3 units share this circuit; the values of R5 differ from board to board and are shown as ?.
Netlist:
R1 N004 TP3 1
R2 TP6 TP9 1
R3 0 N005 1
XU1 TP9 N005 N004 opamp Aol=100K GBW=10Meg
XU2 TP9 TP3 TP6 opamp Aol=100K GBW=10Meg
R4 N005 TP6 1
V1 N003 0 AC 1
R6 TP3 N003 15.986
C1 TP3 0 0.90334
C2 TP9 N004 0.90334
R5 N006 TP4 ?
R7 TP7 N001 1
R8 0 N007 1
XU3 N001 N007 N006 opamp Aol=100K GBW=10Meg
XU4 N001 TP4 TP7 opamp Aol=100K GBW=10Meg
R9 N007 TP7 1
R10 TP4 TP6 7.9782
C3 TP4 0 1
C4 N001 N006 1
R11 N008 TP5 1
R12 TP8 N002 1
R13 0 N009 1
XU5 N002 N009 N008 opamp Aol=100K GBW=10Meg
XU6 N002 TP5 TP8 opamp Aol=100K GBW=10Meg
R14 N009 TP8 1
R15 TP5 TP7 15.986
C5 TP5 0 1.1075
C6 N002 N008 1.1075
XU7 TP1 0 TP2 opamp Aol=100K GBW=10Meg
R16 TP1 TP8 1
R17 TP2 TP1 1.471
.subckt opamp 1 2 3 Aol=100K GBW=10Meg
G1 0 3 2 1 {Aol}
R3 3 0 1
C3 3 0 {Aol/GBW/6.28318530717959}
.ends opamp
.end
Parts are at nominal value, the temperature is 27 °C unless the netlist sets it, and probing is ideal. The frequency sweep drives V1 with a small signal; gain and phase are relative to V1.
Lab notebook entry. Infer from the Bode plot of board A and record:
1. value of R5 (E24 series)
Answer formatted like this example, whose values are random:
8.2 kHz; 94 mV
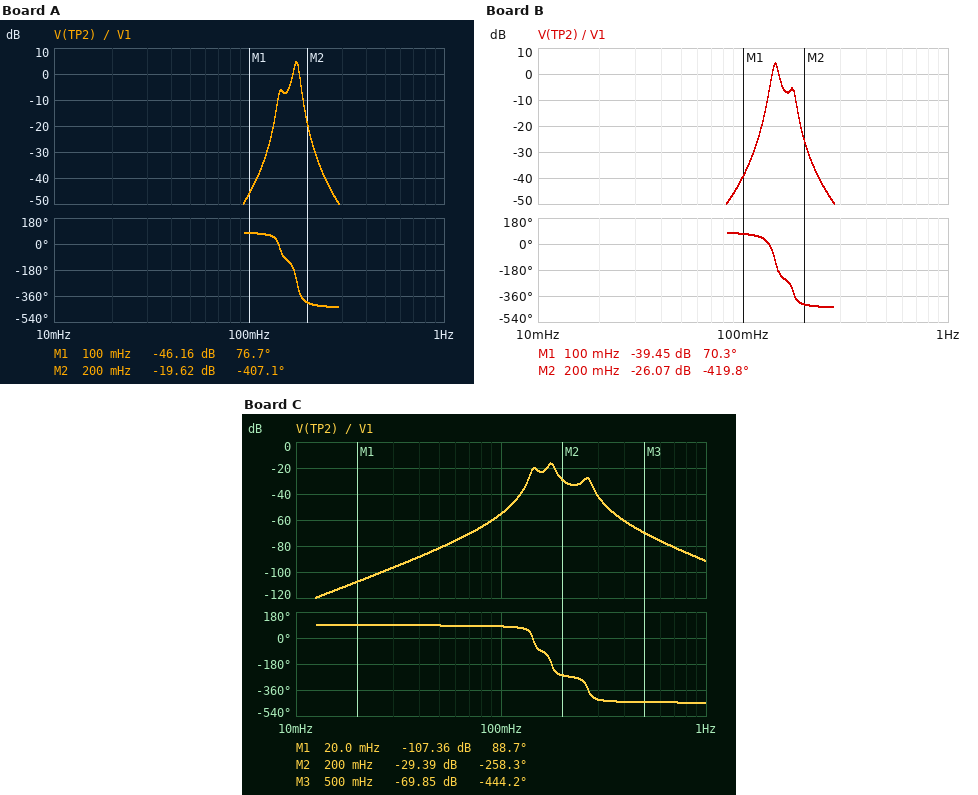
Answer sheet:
0.82 Ω
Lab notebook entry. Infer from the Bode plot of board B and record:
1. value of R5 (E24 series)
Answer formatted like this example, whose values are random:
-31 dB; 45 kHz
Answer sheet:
1.3 Ω
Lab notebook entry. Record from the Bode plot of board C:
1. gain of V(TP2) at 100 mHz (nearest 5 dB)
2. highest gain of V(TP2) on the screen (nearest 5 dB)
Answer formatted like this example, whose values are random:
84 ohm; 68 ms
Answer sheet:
-55 dB; -15 dB
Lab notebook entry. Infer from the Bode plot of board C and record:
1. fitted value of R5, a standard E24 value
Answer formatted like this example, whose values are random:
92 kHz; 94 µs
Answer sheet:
0.36 Ω
